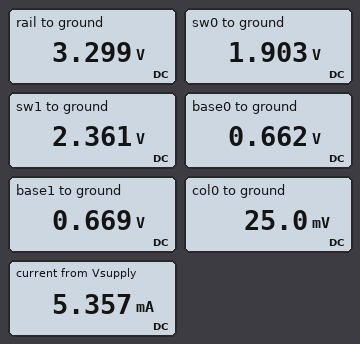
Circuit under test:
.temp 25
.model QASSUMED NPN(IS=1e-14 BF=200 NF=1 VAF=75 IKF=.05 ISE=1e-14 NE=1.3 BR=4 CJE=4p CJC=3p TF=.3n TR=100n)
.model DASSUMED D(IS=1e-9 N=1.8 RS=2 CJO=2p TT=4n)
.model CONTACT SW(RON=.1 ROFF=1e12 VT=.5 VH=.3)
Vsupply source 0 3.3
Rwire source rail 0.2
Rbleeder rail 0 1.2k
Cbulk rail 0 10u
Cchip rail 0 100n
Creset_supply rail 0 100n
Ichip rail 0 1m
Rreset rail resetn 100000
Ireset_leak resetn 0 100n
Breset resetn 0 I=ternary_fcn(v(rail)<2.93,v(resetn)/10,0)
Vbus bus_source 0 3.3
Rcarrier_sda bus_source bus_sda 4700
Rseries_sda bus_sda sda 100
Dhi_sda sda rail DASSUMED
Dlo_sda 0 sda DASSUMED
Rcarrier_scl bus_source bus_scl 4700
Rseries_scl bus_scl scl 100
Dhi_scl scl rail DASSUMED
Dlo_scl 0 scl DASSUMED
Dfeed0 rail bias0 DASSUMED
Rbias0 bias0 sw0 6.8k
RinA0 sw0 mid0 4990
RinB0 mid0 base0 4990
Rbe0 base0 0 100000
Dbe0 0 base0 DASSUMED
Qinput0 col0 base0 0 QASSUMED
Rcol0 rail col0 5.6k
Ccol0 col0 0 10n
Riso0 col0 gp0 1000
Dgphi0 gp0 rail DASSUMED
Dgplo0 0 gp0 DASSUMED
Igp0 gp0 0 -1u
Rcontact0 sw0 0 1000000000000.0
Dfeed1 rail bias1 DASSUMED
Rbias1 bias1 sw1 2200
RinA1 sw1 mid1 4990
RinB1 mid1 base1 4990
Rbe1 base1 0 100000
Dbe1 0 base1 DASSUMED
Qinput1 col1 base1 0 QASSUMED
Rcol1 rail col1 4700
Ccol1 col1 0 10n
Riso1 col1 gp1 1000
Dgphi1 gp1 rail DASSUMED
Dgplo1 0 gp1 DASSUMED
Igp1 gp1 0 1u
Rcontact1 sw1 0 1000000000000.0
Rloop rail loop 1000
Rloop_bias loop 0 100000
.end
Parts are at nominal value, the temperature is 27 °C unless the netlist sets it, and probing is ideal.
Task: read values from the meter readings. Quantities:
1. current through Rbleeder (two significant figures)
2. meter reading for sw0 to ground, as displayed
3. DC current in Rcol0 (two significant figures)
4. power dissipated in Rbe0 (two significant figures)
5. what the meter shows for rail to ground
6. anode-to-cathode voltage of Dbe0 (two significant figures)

2.7 mA
1.903 V
580 µA
4.4 µW
3.299 V
-660 mV
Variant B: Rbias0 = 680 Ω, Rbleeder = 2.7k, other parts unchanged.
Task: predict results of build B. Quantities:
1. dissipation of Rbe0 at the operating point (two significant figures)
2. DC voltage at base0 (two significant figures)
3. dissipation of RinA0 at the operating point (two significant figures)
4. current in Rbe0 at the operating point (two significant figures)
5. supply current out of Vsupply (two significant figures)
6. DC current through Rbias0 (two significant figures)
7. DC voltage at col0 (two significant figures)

4.5 µW
670 mV
190 µW
6.7 µA
3.9 mA
190 µA
19 mV
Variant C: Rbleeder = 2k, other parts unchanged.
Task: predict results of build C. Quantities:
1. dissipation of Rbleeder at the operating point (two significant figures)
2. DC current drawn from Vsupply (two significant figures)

5.4 mW
4.3 mA
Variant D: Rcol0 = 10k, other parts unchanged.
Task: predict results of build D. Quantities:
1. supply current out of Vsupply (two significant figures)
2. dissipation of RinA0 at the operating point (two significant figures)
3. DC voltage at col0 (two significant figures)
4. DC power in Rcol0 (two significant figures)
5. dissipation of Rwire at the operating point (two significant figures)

5.1 mA
78 µW
18 mV
1.1 mW
5.2 µW
